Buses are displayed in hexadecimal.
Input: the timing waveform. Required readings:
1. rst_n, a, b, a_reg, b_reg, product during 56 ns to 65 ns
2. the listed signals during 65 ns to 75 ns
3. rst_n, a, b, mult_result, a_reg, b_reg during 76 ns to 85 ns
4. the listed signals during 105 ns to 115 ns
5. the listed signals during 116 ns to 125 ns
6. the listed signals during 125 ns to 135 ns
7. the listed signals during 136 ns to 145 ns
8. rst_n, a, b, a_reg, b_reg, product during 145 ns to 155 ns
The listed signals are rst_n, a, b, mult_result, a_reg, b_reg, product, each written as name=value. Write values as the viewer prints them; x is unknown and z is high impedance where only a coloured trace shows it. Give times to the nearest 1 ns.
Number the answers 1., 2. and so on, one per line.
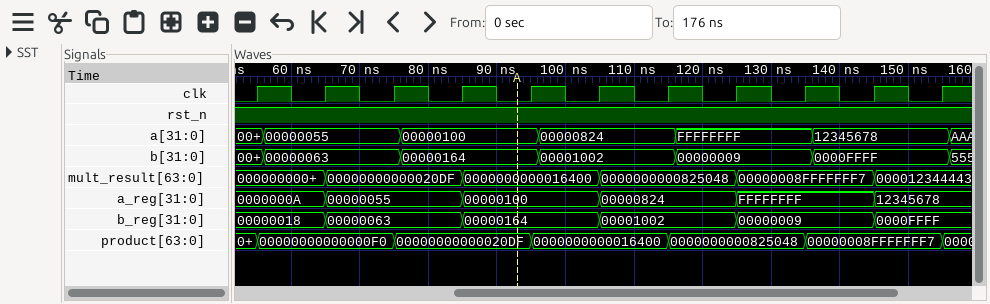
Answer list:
1. rst_n=1, a=00000055, b=00000063, a_reg=0000000A, b_reg=00000018, product=00000000000000F0
2. rst_n=1, a=00000055, b=00000063, mult_result=00000000000020DF, a_reg=00000055, b_reg=00000063, product=00000000000000F0
3. rst_n=1, a=00000100, b=00000164, mult_result=00000000000020DF, a_reg=00000055, b_reg=00000063
4. rst_n=1, a=00000824, b=00001002, mult_result=0000000000825048, a_reg=00000824, b_reg=00001002, product=0000000000016400
5. rst_n=1, a=FFFFFFFF, b=00000009, mult_result=0000000000825048, a_reg=00000824, b_reg=00001002, product=0000000000825048
6. rst_n=1, a=FFFFFFFF, b=00000009, mult_result=00000008FFFFFFF7, a_reg=FFFFFFFF, b_reg=00000009, product=0000000000825048
7. rst_n=1, a=12345678, b=0000FFFF, mult_result=00000008FFFFFFF7, a_reg=FFFFFFFF, b_reg=00000009, product=00000008FFFFFFF7
8. rst_n=1, a=12345678, b=0000FFFF, a_reg=12345678, b_reg=0000FFFF, product=00000008FFFFFFF7
